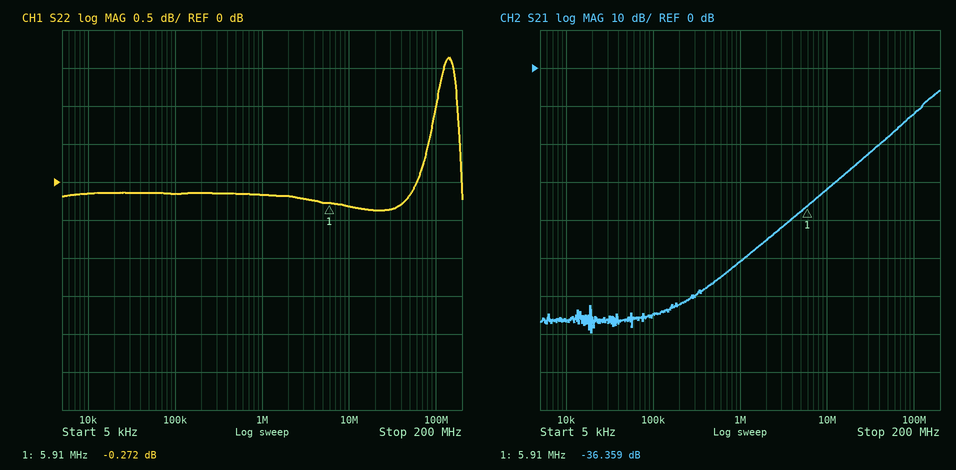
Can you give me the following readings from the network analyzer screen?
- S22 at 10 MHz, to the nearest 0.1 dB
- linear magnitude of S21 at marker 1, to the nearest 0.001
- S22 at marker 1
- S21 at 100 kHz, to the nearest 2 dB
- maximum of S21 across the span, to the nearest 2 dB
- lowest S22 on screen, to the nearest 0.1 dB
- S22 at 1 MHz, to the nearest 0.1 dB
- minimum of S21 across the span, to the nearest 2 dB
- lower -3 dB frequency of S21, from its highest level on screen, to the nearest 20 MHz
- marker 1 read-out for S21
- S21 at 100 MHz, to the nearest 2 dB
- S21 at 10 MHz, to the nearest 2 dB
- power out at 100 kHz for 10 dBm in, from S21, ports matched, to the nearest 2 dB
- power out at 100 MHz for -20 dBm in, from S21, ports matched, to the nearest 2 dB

-0.3 dB
0.015
-0.272 dB
-64 dB
-6 dB
-0.4 dB
-0.2 dB
-70 dB
140 MHz
-36.359 dB
-12 dB
-32 dB
-54 dBm
-32 dBm
